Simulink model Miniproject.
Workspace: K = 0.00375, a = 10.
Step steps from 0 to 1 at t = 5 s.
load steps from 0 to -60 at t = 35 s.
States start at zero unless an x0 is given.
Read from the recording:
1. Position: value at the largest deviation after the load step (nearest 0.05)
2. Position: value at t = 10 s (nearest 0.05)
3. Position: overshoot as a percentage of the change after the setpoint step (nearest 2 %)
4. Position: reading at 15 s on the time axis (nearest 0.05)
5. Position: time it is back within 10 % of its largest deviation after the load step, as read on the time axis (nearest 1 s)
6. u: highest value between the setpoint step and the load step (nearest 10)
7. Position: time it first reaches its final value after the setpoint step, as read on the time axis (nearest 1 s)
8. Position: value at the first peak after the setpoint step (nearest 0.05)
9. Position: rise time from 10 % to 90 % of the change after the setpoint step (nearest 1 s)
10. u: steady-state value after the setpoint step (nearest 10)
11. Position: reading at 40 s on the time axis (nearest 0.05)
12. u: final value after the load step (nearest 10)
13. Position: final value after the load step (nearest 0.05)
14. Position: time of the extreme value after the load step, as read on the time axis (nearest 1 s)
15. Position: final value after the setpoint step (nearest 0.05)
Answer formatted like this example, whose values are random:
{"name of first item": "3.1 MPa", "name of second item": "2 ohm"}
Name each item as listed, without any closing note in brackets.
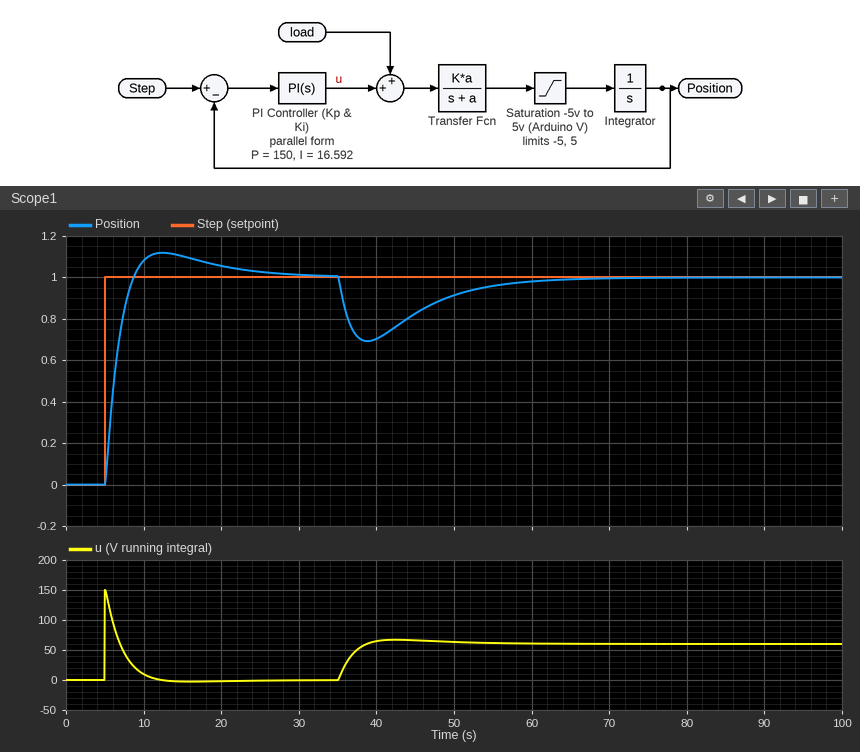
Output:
{"Position: value at the largest deviation after the load step": "0.70", "Position: value at t = 10 s": "1.10", "Position: overshoot as a percentage of the change after the setpoint step": "12 %", "Position: reading at 15 s on the time axis": "1.10", "Position: time it is back within 10 % of its largest deviation after the load step, as read on the time axis": "57 s", "u: highest value between the setpoint step and the load step": "150", "Position: time it first reaches its final value after the setpoint step, as read on the time axis": "9 s", "Position: value at the first peak after the setpoint step": "1.10", "Position: rise time from 10 % to 90 % of the change after the setpoint step": "3 s", "u: steady-state value after the setpoint step": "0", "Position: reading at 40 s on the time axis": "0.70", "u: final value after the load step": "60", "Position: final value after the load step": "1.00", "Position: time of the extreme value after the load step, as read on the time axis": "39 s", "Position: final value after the setpoint step": "1.00"}
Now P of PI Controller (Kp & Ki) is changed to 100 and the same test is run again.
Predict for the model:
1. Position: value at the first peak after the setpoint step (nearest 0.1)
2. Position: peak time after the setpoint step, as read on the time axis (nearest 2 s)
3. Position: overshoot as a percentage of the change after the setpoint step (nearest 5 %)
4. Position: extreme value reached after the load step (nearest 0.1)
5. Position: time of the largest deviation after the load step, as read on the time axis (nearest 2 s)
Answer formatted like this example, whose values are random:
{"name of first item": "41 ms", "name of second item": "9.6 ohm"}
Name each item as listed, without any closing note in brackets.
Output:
{"Position: value at the first peak after the setpoint step": "1.2", "Position: peak time after the setpoint step, as read on the time axis": "14 s", "Position: overshoot as a percentage of the change after the setpoint step": "20 %", "Position: extreme value reached after the load step": "0.6", "Position: time of the largest deviation after the load step, as read on the time axis": "40 s"}
